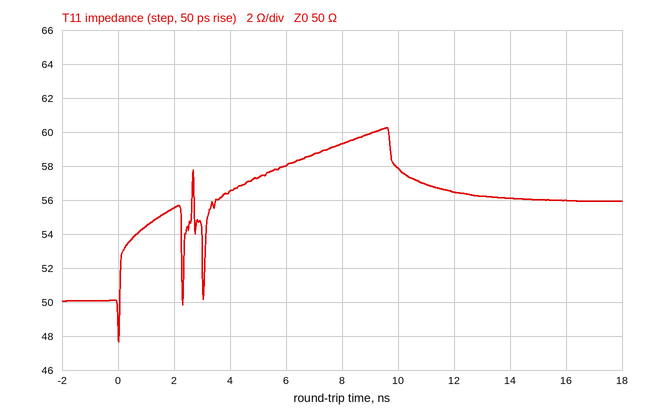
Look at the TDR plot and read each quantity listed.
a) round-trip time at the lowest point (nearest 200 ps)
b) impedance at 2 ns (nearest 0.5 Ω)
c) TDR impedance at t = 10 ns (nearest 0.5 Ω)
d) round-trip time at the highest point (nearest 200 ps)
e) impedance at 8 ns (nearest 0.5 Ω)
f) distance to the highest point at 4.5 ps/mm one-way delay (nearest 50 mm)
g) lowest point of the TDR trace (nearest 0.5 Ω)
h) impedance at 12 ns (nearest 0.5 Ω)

0.0 ns
55.5 Ω
58.0 Ω
9.6 ns
59.5 Ω
1.05 m
47.5 Ω
56.5 Ω
